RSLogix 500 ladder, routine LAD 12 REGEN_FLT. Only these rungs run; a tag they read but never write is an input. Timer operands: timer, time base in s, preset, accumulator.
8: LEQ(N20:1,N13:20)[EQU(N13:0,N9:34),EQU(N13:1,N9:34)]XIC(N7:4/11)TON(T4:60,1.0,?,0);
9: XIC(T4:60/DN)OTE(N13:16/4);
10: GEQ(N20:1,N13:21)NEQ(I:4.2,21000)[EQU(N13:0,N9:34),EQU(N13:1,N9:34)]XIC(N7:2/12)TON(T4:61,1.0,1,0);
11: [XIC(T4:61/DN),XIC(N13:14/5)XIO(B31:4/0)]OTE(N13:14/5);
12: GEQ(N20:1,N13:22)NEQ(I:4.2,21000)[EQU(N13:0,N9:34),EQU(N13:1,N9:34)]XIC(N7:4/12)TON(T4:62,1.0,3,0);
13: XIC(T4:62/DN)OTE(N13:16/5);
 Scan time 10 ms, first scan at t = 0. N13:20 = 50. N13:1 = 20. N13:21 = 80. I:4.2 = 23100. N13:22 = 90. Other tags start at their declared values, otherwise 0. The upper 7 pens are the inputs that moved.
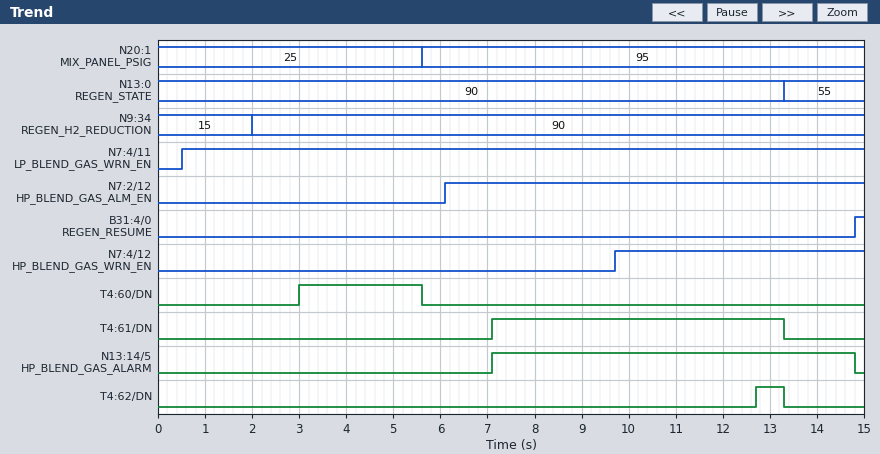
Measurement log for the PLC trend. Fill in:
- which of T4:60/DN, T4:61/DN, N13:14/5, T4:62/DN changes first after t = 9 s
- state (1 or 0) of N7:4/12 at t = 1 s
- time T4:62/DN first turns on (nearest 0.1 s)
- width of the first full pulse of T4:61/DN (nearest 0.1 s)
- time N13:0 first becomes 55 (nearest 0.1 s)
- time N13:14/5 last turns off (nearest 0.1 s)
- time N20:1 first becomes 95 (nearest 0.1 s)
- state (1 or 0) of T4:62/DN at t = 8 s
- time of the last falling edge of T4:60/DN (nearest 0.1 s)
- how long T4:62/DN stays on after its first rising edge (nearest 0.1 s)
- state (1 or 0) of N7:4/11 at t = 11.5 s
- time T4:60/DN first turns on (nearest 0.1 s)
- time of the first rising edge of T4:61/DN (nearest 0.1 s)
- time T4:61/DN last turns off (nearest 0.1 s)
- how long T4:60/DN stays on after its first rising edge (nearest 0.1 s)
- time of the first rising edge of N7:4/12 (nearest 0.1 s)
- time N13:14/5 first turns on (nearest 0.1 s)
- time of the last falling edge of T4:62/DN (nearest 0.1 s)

T4:62/DN
0
12.7 s
6.2 s
13.3 s
14.8 s
5.6 s
0
5.6 s
0.6 s
1
3.0 s
7.1 s
13.3 s
2.6 s
9.7 s
7.1 s
13.3 s
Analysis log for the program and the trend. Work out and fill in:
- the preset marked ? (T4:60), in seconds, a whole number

1 s
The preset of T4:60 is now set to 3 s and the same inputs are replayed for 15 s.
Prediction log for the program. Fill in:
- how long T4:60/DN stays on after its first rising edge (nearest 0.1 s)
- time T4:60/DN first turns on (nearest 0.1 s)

0.6 s
5.0 s
